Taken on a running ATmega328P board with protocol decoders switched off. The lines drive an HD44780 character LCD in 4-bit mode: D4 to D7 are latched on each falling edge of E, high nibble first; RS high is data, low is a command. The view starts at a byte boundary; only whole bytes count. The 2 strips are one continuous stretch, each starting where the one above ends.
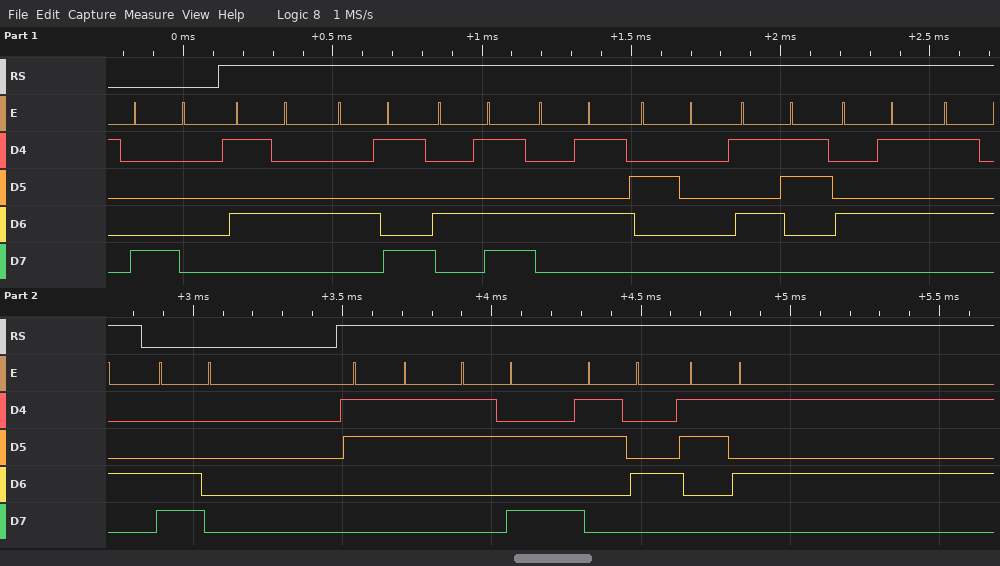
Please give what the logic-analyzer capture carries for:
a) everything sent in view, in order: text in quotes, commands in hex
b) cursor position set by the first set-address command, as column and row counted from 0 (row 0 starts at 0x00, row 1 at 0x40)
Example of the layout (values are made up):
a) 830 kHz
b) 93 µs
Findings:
a) 0x80 "TIME SET" 0xC0 "3:45"
b) column 0, row 0
